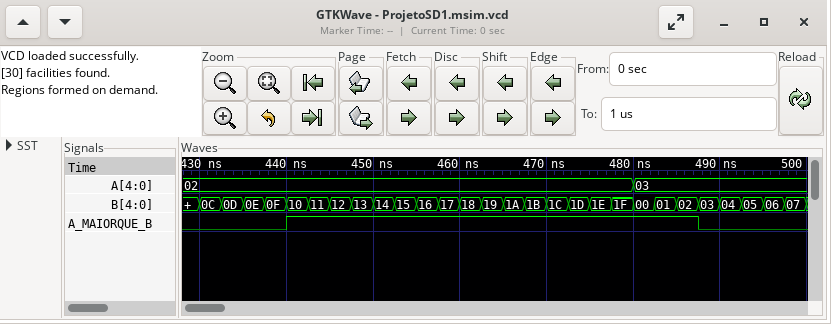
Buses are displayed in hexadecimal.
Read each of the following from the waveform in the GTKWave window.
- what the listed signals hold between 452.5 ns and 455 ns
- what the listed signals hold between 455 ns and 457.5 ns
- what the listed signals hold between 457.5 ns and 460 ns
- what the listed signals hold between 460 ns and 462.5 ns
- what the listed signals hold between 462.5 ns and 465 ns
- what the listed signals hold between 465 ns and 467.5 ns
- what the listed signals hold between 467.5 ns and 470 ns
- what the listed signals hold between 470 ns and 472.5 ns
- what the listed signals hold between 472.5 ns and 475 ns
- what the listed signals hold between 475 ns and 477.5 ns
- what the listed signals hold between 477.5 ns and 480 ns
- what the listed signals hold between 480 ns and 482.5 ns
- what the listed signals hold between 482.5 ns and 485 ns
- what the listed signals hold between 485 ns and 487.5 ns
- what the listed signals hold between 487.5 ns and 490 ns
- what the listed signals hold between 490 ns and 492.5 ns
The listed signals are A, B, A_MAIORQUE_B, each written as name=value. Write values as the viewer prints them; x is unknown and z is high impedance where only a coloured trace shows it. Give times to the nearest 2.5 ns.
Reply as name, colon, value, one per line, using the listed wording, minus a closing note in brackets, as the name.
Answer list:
what the listed signals hold between 452.5 ns and 455 ns: A=02, B=15, A_MAIORQUE_B=1
what the listed signals hold between 455 ns and 457.5 ns: A=02, B=16, A_MAIORQUE_B=1
what the listed signals hold between 457.5 ns and 460 ns: A=02, B=17, A_MAIORQUE_B=1
what the listed signals hold between 460 ns and 462.5 ns: A=02, B=18, A_MAIORQUE_B=1
what the listed signals hold between 462.5 ns and 465 ns: A=02, B=19, A_MAIORQUE_B=1
what the listed signals hold between 465 ns and 467.5 ns: A=02, B=1A, A_MAIORQUE_B=1
what the listed signals hold between 467.5 ns and 470 ns: A=02, B=1B, A_MAIORQUE_B=1
what the listed signals hold between 470 ns and 472.5 ns: A=02, B=1C, A_MAIORQUE_B=1
what the listed signals hold between 472.5 ns and 475 ns: A=02, B=1D, A_MAIORQUE_B=1
what the listed signals hold between 475 ns and 477.5 ns: A=02, B=1E, A_MAIORQUE_B=1
what the listed signals hold between 477.5 ns and 480 ns: A=02, B=1F, A_MAIORQUE_B=1
what the listed signals hold between 480 ns and 482.5 ns: A=03, B=00, A_MAIORQUE_B=1
what the listed signals hold between 482.5 ns and 485 ns: A=03, B=01, A_MAIORQUE_B=1
what the listed signals hold between 485 ns and 487.5 ns: A=03, B=02, A_MAIORQUE_B=1
what the listed signals hold between 487.5 ns and 490 ns: A=03, B=03, A_MAIORQUE_B=0
what the listed signals hold between 490 ns and 492.5 ns: A=03, B=04, A_MAIORQUE_B=0
